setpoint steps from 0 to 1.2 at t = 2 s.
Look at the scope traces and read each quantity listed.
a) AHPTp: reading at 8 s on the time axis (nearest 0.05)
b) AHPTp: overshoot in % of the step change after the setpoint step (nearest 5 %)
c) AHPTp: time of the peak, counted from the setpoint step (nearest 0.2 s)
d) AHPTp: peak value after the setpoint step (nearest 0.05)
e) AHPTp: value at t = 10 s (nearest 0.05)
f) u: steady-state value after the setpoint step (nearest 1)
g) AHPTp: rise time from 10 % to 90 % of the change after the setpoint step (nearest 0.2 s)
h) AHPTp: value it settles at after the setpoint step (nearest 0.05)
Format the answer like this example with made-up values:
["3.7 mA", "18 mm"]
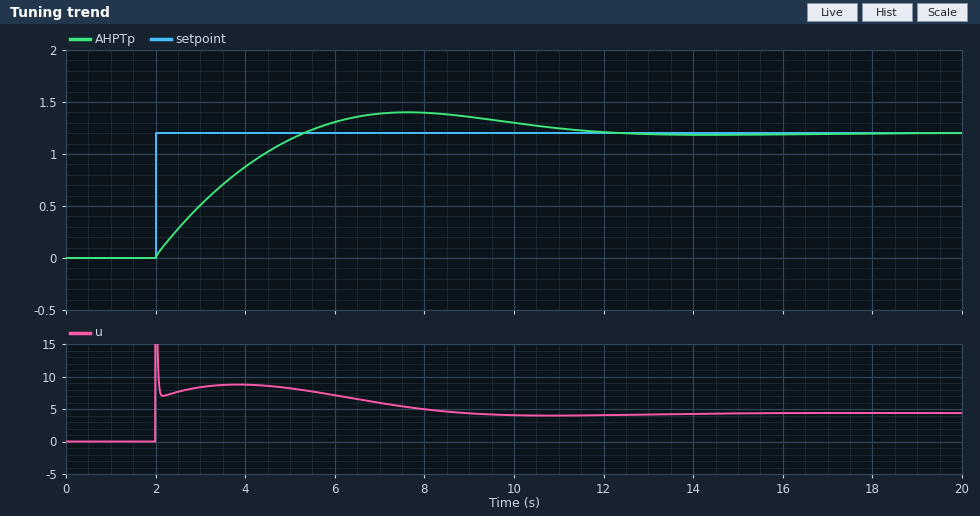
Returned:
["1.40", "15 %", "5.6 s", "1.40", "1.30", "4", "2.6 s", "1.20"]
